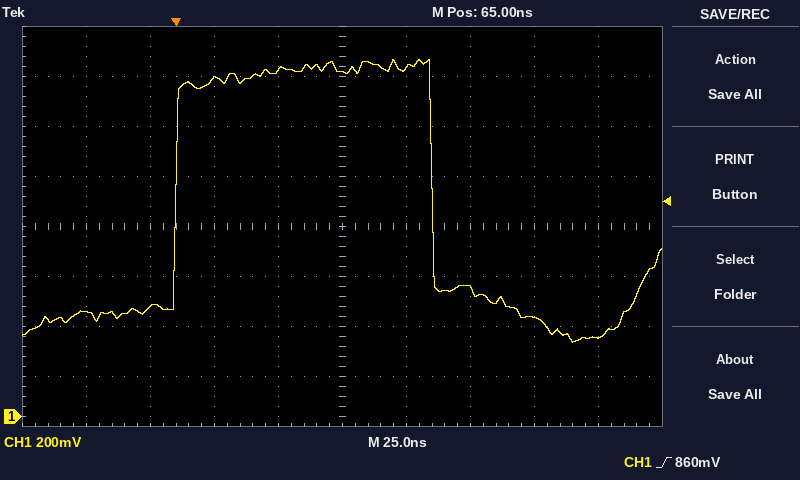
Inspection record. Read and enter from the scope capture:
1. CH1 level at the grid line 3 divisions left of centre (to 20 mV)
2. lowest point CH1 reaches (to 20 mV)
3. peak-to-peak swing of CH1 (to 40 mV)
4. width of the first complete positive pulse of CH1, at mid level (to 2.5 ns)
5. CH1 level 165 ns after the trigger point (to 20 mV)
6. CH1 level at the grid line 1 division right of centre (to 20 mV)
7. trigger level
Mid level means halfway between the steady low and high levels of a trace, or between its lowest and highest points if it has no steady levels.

440 mV
300 mV
1.12 V
100.0 ns
320 mV
1.40 V
860 mV
